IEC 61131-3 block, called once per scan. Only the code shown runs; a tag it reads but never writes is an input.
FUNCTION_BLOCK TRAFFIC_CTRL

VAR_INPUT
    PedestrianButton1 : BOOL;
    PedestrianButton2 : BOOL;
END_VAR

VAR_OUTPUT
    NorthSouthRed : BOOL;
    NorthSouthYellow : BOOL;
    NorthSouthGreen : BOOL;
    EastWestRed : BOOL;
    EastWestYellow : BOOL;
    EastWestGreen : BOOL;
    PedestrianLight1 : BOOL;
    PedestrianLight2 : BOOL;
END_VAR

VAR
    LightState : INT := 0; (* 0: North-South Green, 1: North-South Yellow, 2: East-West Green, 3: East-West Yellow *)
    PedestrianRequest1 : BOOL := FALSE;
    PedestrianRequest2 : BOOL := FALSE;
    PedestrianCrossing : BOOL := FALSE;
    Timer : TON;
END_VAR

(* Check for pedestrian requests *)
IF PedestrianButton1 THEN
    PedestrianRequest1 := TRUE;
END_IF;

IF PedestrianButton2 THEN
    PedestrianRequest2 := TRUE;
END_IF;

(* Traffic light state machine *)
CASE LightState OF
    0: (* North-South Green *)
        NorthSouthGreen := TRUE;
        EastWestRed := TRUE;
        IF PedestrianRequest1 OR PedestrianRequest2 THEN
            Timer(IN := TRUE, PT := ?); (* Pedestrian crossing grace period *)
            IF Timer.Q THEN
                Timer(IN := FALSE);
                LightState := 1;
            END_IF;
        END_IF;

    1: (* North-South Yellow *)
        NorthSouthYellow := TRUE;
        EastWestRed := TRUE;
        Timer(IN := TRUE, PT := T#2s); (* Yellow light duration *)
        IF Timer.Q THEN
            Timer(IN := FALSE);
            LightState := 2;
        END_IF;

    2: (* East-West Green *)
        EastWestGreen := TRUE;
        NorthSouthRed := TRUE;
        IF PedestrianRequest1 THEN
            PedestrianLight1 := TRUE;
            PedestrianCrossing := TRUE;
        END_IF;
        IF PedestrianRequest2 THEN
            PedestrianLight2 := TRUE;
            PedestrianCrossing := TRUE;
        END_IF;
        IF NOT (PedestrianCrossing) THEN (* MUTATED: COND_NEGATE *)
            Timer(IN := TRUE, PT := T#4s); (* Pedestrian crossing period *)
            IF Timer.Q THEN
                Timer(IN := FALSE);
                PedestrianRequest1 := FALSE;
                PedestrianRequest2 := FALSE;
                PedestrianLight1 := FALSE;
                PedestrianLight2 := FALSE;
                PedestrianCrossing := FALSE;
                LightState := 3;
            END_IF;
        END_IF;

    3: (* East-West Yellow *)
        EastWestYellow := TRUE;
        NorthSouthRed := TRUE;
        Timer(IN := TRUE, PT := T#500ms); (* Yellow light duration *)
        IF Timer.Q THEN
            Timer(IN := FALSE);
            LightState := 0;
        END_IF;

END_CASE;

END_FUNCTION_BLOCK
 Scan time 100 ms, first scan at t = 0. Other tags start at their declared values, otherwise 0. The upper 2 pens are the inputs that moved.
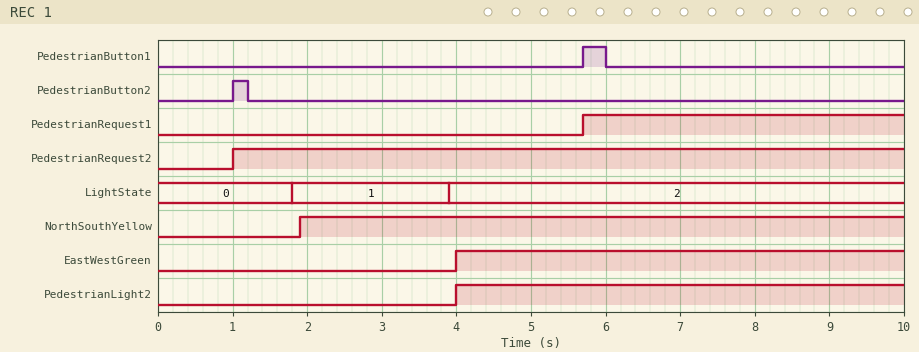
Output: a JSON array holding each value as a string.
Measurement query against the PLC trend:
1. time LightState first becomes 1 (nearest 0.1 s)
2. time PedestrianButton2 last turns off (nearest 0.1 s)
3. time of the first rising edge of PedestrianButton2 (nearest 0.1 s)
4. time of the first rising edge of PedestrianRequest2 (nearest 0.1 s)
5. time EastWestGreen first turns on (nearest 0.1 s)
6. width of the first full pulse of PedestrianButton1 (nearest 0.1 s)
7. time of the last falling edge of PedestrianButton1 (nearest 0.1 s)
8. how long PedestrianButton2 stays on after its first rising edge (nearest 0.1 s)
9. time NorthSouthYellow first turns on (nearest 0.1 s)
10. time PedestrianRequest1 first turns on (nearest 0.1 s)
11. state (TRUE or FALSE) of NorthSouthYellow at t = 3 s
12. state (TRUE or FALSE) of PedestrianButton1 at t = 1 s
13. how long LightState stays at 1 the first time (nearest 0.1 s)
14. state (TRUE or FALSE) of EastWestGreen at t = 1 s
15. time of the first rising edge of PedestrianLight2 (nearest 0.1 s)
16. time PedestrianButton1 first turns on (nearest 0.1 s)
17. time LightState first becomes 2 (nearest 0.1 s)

["1.8 s", "1.2 s", "1.0 s", "1.0 s", "4.0 s", "0.3 s", "6.0 s", "0.2 s", "1.9 s", "5.7 s", "TRUE", "FALSE", "2.1 s", "FALSE", "4.0 s", "5.7 s", "3.9 s"]
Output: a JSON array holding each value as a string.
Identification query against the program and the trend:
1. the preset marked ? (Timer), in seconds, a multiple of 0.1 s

["0.8 s"]
